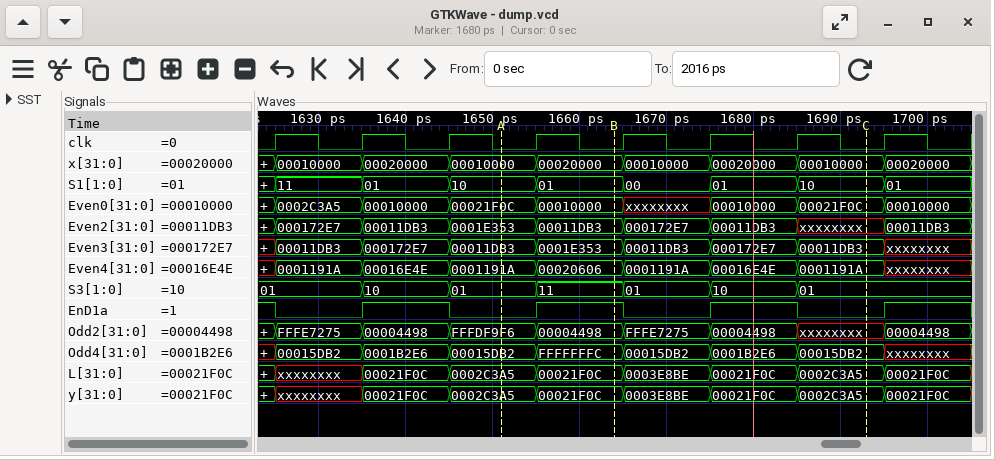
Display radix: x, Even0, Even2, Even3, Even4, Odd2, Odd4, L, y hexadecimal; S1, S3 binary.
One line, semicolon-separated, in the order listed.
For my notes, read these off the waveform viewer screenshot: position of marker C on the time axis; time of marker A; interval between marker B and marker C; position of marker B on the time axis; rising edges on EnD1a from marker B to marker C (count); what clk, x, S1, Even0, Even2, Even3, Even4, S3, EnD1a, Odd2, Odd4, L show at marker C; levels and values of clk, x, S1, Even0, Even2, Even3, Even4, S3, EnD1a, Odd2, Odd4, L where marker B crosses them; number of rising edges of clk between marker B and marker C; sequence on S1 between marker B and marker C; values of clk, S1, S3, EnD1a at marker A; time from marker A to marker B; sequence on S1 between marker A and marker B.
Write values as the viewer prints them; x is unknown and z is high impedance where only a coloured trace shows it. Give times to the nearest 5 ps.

1695 ps; 1650 ps; 30 ps; 1665 ps; 1; clk=0, x=00010000, S1=10, Even0=00021F0C, Even2=xxxxxxxx, Even3=00011DB3, Even4=0001191A, S3=01, EnD1a=0, Odd2=xxxxxxxx, Odd4=00015DB2, L=0002C3A5; clk=0, x=00020000, S1=01, Even0=00010000, Even2=00011DB3, Even3=0001E353, Even4=00020606, S3=11, EnD1a=1, Odd2=00004498, Odd4=FFFFFFFC, L=00021F0C; 3; 01, 00, 01, 10; clk=0, S1=10, S3=01, EnD1a=0; 15 ps; 10, 01
